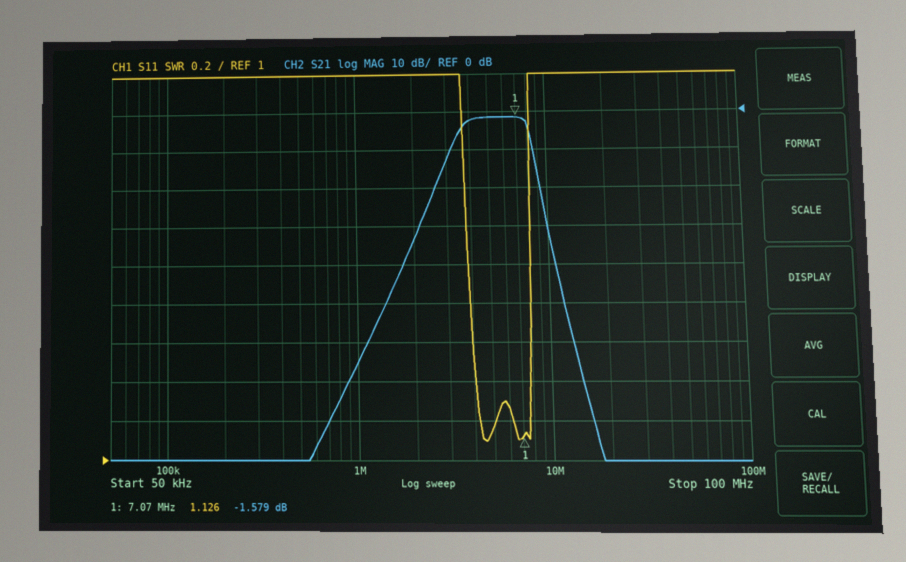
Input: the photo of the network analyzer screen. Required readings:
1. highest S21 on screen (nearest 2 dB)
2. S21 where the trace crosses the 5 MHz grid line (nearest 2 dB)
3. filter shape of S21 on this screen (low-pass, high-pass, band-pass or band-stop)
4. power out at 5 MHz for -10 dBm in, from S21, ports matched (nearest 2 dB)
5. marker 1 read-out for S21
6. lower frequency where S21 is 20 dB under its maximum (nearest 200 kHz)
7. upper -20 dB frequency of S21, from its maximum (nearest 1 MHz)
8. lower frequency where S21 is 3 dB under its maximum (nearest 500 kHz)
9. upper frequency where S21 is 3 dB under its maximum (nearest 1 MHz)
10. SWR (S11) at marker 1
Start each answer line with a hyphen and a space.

- -2 dB
- -2 dB
- band-pass
- -12 dBm
- -1.579 dB
- 2.6 MHz
- 9 MHz
- 3.5 MHz
- 8 MHz
- 1.126
